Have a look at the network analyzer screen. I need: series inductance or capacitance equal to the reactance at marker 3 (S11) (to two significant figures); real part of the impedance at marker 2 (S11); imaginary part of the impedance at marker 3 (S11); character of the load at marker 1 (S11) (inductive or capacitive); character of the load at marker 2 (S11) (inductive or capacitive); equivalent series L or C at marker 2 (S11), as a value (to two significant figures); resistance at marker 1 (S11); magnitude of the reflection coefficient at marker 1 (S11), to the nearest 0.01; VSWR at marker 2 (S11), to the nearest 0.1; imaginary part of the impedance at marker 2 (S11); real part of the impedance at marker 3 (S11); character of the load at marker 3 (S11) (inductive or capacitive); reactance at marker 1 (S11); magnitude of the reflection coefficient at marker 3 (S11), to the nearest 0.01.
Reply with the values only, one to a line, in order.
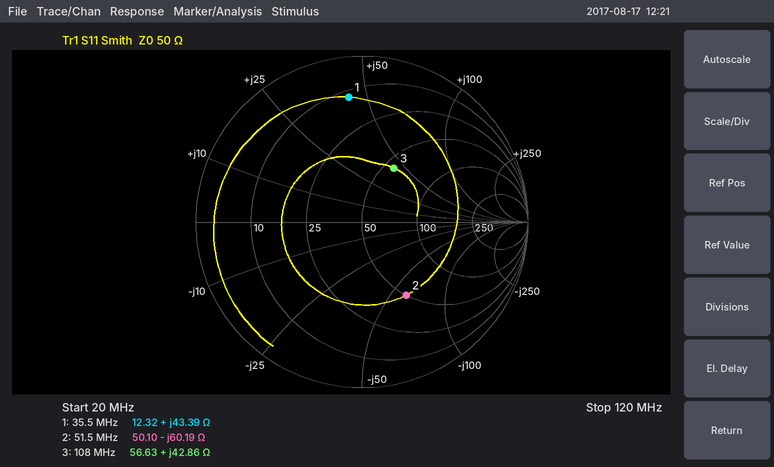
63 nH
50.10 Ω
+42.86 Ω
inductive
capacitive
51 pF
12.32 Ω
0.76
3.1
-60.19 Ω
56.63 Ω
inductive
+43.39 Ω
0.38
